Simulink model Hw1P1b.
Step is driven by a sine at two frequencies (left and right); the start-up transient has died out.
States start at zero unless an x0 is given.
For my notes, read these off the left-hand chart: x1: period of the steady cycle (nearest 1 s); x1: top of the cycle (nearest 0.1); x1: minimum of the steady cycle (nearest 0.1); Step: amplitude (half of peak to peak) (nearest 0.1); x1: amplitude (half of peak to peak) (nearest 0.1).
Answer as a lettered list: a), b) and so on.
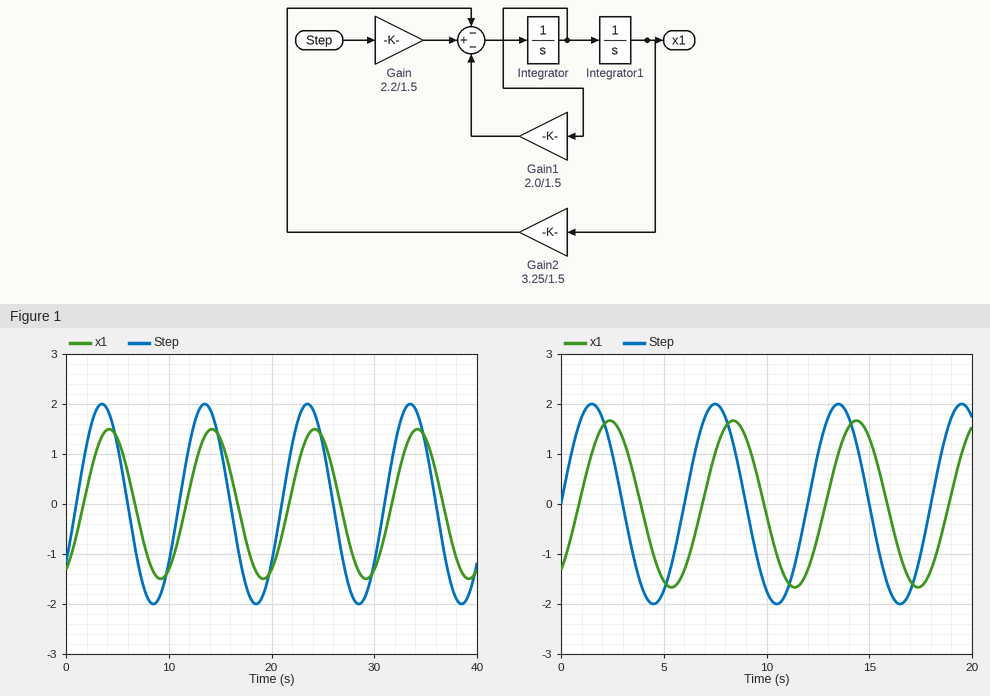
a) 10 s
b) 1.5
c) -1.5
d) 2.0
e) 1.5
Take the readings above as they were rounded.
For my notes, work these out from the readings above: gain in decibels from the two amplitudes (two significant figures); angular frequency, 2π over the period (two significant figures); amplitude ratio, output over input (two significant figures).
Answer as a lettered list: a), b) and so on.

a) -2.5 dB
b) 0.63 rad/s
c) 0.75
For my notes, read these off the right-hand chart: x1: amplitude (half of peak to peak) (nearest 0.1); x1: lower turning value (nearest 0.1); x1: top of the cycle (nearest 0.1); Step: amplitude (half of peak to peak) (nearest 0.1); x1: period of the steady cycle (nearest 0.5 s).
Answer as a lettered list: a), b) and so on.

a) 1.7
b) -1.7
c) 1.7
d) 2.0
e) 6.0 s
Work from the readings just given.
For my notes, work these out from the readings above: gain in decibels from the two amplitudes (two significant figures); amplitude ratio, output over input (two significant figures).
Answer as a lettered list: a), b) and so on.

a) -1.4 dB
b) 0.85
